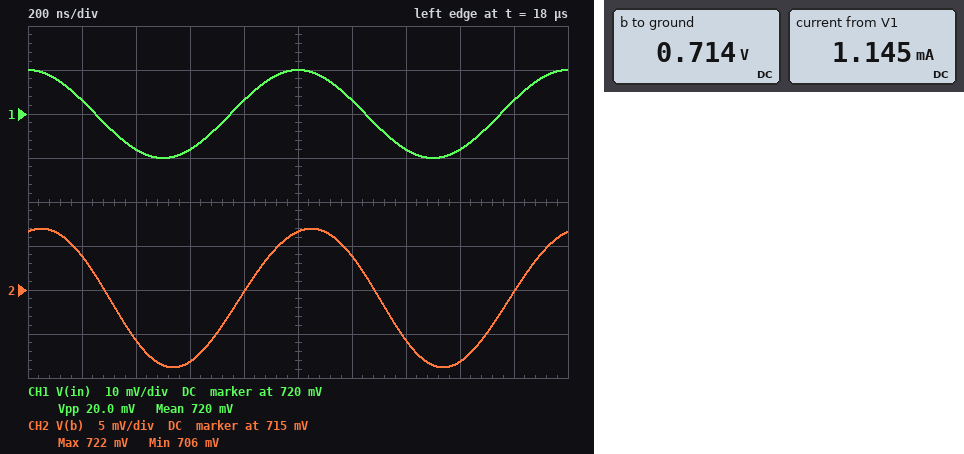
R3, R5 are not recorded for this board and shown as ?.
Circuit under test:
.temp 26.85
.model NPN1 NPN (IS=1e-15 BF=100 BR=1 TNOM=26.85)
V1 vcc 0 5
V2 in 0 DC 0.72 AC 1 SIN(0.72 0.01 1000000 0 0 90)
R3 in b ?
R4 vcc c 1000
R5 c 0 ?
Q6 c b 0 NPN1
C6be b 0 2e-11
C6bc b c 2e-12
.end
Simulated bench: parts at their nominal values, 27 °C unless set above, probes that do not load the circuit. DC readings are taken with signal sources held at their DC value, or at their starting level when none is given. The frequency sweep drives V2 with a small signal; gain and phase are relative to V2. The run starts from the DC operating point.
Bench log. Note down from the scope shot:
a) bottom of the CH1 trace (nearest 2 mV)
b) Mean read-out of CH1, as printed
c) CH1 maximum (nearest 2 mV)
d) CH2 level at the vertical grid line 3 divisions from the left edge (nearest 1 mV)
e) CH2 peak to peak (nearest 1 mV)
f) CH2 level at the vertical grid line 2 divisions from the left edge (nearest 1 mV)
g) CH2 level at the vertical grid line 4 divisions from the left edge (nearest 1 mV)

710 mV
720 mV
730 mV
707 mV
16 mV
709 mV
715 mV
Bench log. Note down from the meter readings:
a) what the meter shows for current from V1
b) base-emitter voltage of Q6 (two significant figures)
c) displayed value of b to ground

1.145 mA
710 mV
0.714 V
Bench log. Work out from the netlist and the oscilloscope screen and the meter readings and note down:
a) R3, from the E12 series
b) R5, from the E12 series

560 Ω
27 kΩ
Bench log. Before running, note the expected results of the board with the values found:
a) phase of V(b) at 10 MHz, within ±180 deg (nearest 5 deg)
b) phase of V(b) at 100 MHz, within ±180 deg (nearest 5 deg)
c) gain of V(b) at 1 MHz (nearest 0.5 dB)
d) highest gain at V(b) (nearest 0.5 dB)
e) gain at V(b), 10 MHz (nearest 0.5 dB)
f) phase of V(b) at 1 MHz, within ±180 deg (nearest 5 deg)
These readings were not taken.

-65 deg
-50 deg
-2.0 dB
-1.5 dB
-11.5 dB
-15 deg
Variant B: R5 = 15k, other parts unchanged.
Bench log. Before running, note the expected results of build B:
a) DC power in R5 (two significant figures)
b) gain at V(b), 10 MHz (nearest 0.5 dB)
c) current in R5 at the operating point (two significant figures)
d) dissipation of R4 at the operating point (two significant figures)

940 µW
-11.0 dB
250 µA
1.6 mW
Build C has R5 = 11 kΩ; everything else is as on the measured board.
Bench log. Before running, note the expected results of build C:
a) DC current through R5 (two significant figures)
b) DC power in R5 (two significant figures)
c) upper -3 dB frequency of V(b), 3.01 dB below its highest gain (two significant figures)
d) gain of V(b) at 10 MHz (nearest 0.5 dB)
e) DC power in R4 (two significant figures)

330 µA
1.2 mW
3.6 MHz
-11.0 dB
1.8 mW
